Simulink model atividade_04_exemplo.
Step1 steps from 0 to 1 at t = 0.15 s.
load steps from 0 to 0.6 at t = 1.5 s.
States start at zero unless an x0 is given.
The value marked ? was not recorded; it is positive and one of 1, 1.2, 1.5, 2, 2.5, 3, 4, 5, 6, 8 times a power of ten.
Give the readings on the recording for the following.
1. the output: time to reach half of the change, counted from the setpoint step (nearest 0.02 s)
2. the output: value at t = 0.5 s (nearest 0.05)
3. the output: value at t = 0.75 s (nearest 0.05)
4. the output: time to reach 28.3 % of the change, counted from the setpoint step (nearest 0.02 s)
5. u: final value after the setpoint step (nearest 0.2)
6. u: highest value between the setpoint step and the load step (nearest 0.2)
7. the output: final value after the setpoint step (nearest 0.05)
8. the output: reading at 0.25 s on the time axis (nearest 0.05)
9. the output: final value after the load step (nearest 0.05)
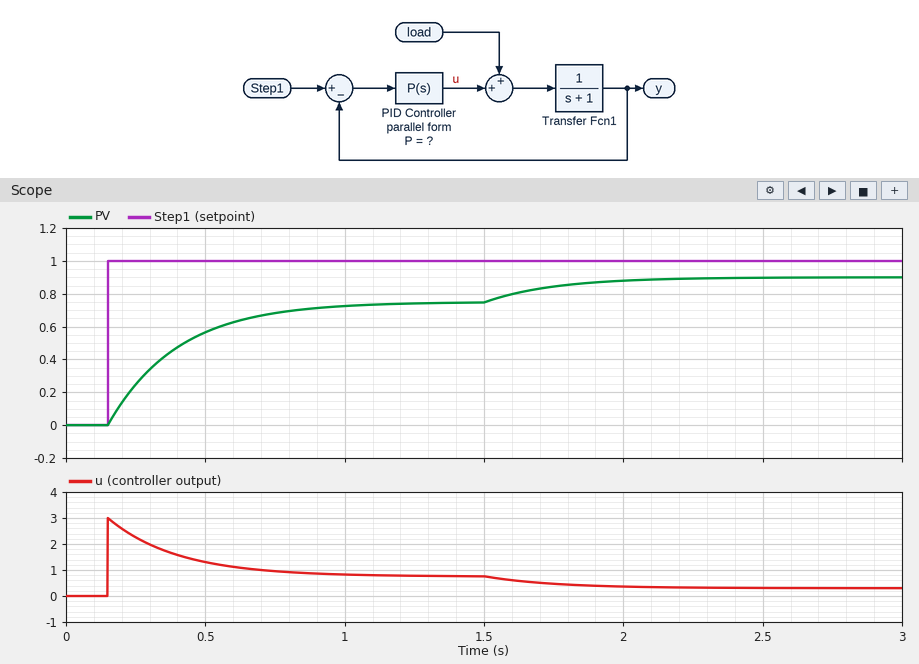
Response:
0.18 s
0.55
0.70
0.08 s
0.8
3.0
0.75
0.25
0.90
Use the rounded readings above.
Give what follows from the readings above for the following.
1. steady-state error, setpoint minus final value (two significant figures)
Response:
0.25
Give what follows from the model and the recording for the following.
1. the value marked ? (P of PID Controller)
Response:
3
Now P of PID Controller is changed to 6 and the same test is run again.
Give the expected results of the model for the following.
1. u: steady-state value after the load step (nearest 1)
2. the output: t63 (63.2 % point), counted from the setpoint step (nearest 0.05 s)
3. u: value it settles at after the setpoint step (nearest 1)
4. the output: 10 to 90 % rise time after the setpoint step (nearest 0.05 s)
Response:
0
0.15 s
1
0.30 s
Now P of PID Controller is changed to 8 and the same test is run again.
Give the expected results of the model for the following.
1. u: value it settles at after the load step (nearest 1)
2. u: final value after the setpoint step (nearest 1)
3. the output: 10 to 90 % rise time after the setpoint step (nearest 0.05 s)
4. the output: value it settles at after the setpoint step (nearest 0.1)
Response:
0
1
0.25 s
0.9
